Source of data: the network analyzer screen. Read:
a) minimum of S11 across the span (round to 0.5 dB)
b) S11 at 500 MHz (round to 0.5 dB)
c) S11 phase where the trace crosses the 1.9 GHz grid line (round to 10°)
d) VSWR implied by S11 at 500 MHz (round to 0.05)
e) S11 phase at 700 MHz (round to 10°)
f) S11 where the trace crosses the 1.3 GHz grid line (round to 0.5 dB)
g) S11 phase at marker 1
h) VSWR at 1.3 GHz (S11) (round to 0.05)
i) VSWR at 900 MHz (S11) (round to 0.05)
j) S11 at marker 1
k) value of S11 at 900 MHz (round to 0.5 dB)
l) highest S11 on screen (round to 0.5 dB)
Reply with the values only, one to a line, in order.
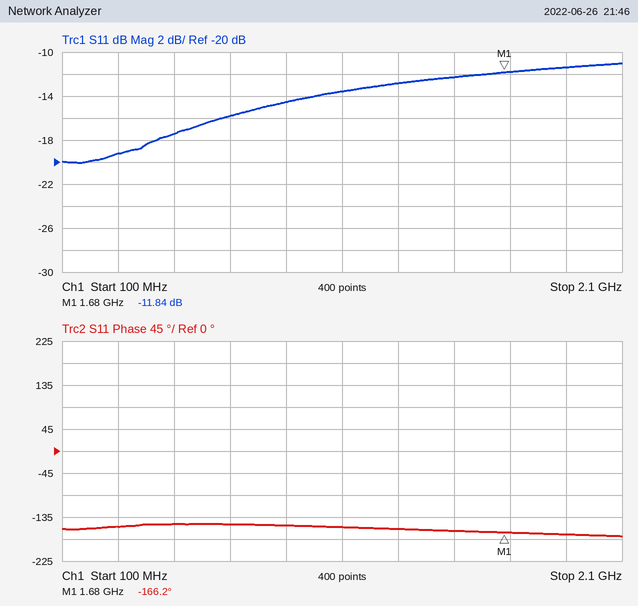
-20.0 dB
-17.5 dB
-170°
1.30
-150°
-13.0 dB
-166.2°
1.60
1.45
-11.84 dB
-14.5 dB
-11.0 dB
